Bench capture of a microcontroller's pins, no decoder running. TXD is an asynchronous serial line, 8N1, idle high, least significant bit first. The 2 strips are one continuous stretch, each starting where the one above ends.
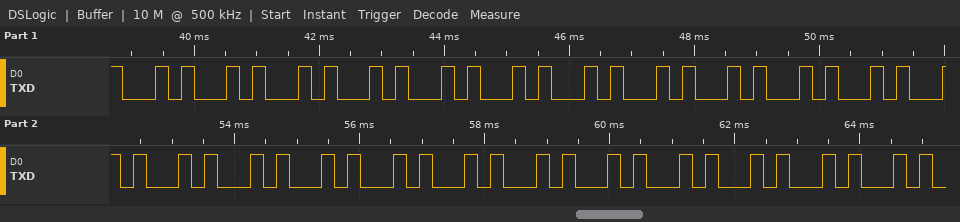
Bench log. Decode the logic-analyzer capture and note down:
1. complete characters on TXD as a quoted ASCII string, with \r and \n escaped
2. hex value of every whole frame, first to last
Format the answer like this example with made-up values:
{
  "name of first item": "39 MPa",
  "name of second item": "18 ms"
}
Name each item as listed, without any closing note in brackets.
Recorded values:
{
  "complete characters on TXD as a quoted ASCII string, with \\r and \\n escaped": "\"00000000000000000000000\"",
  "hex value of every whole frame, first to last": "30 30 30 30 30 30 30 30 30 30 30 30 30 30 30 30 30 30 30 30 30 30 30"
}
